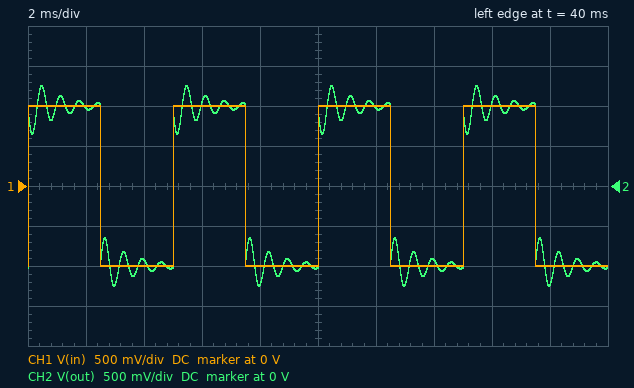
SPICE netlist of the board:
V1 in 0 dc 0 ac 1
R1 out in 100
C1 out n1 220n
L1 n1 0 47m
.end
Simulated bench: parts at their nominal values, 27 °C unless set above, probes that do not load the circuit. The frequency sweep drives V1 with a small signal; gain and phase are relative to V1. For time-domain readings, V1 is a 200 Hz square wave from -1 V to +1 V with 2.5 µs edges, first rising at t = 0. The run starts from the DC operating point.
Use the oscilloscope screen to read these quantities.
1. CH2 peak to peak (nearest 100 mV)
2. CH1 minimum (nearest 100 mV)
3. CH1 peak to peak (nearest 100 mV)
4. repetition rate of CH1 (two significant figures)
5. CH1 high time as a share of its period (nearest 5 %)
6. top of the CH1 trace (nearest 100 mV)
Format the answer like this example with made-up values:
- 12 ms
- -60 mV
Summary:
- 2.5 V
- -1.0 V
- 2.0 V
- 200 Hz
- 50 %
- 1.0 V
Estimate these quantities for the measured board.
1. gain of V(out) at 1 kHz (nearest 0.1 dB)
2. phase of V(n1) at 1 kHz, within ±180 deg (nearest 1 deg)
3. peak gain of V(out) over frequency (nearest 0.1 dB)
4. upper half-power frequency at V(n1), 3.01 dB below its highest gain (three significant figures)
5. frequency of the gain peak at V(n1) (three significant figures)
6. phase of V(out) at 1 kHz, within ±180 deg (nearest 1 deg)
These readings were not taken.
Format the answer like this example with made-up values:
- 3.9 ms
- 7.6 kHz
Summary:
- -0.2 dB
- 167 deg
- 0 dB
- 1.79 kHz
- 1.58 kHz
- -13 deg
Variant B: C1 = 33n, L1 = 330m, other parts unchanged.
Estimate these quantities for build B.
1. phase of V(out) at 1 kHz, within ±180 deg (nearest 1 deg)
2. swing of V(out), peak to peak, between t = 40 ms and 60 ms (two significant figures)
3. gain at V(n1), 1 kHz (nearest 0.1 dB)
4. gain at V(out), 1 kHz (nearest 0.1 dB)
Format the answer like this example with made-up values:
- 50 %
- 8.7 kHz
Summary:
- -2 deg
- 2.1 V
- -2.5 dB
- 0 dB
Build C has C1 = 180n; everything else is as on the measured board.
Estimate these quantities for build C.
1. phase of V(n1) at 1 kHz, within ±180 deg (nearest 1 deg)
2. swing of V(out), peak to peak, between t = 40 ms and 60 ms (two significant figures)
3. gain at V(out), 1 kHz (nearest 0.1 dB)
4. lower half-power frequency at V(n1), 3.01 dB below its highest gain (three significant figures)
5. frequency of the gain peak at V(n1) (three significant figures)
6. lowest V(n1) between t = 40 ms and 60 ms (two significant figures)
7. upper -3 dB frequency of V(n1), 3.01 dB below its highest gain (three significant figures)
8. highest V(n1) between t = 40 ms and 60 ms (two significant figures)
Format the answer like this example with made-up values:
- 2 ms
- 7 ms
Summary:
- 170 deg
- 2.5 V
- -0.1 dB
- 1.60 kHz
- 1.75 kHz
- -2.0 V
- 1.95 kHz
- 2.0 V
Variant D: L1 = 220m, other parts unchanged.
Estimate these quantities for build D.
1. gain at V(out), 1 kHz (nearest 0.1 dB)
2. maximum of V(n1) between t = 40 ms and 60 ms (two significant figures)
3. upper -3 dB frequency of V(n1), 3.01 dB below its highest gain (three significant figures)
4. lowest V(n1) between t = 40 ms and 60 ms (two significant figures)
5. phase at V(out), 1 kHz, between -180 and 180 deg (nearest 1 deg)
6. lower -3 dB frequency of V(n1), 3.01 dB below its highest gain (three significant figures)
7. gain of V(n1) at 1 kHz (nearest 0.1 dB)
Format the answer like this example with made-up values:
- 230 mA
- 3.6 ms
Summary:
- -0.1 dB
- 1.4 V
- 765 Hz
- -1.4 V
- 9 deg
- 691 Hz
- 6.3 dB
